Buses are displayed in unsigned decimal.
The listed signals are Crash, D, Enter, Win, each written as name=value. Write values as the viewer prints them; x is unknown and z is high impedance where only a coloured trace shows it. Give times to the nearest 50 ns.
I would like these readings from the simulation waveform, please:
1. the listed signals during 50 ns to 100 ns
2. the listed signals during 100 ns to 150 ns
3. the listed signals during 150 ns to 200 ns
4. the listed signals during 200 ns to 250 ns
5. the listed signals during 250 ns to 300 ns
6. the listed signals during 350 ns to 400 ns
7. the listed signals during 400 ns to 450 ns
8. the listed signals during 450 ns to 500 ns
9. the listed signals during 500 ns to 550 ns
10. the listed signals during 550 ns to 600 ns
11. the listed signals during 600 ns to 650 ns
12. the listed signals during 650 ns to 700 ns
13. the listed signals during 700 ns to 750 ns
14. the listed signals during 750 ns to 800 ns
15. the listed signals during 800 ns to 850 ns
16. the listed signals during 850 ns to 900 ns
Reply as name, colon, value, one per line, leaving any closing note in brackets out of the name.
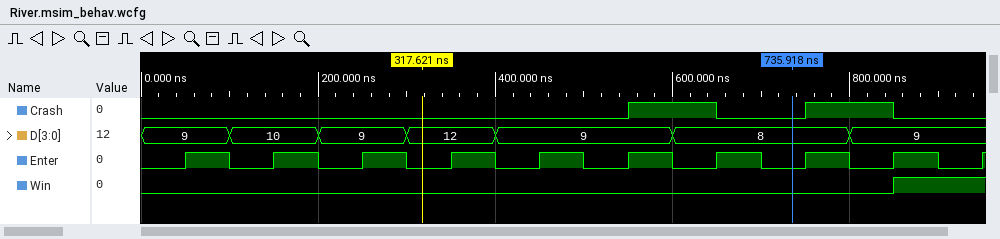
the listed signals during 50 ns to 100 ns: Crash=0, D=9, Enter=1, Win=0
the listed signals during 100 ns to 150 ns: Crash=0, D=10, Enter=0, Win=0
the listed signals during 150 ns to 200 ns: Crash=0, D=10, Enter=1, Win=0
the listed signals during 200 ns to 250 ns: Crash=0, D=9, Enter=0, Win=0
the listed signals during 250 ns to 300 ns: Crash=0, D=9, Enter=1, Win=0
the listed signals during 350 ns to 400 ns: Crash=0, D=12, Enter=1, Win=0
the listed signals during 400 ns to 450 ns: Crash=0, D=9, Enter=0, Win=0
the listed signals during 450 ns to 500 ns: Crash=0, D=9, Enter=1, Win=0
the listed signals during 500 ns to 550 ns: Crash=0, D=9, Enter=0, Win=0
the listed signals during 550 ns to 600 ns: Crash=1, D=9, Enter=1, Win=0
the listed signals during 600 ns to 650 ns: Crash=1, D=8, Enter=0, Win=0
the listed signals during 650 ns to 700 ns: Crash=0, D=8, Enter=1, Win=0
the listed signals during 700 ns to 750 ns: Crash=0, D=8, Enter=0, Win=0
the listed signals during 750 ns to 800 ns: Crash=1, D=8, Enter=1, Win=0
the listed signals during 800 ns to 850 ns: Crash=1, D=9, Enter=0, Win=0
the listed signals during 850 ns to 900 ns: Crash=0, D=9, Enter=1, Win=1
